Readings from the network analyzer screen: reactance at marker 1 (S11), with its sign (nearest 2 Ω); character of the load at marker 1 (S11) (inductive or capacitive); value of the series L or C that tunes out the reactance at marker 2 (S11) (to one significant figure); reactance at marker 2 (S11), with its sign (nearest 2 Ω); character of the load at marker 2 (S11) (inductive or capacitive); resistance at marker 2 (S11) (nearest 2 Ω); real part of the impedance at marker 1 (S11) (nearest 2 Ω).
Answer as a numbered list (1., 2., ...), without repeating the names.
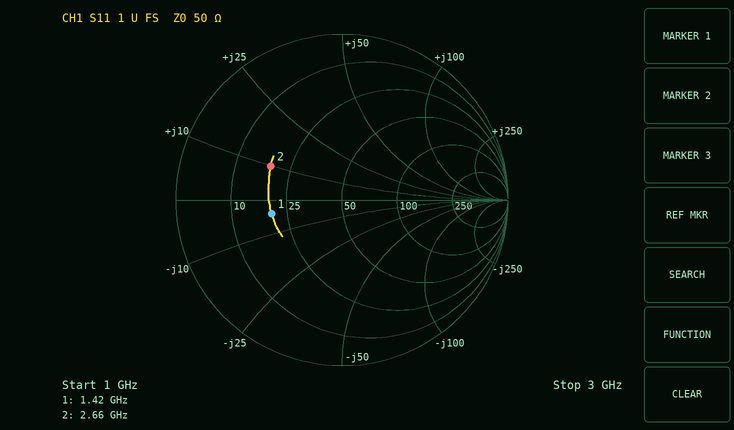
1. -4 Ω
2. capacitive
3. 6 pF
4. +10 Ω
5. inductive
6. 18 Ω
7. 20 Ω
